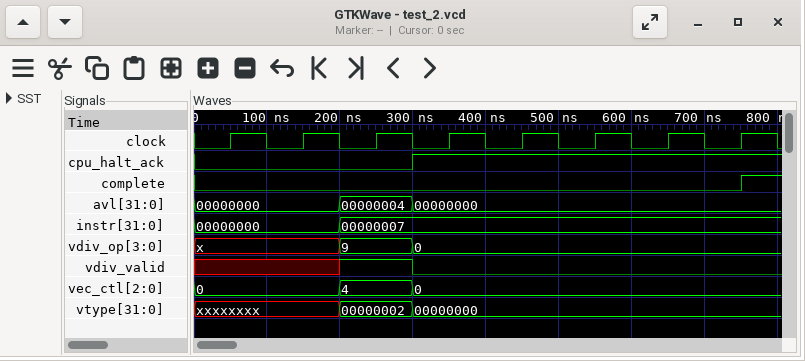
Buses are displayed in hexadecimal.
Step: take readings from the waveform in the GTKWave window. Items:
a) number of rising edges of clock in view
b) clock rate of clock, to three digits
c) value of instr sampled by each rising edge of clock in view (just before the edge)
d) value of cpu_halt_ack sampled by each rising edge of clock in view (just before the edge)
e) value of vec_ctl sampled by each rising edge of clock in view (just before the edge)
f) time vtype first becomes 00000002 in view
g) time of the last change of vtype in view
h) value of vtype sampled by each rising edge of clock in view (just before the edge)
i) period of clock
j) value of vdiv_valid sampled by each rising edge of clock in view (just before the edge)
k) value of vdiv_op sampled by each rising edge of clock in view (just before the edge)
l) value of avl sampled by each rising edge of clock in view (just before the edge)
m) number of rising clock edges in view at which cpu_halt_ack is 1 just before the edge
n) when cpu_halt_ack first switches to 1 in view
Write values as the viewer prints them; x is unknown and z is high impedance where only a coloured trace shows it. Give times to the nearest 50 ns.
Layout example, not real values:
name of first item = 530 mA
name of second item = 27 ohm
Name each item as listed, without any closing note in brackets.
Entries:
number of rising edges of clock in view = 8
clock rate of clock, to three digits = 10.0 MHz
value of instr sampled by each rising edge of clock in view = 00000000, 00000000, 00000007, 00000007, 00000007, 00000007, 00000007, 00000007
value of cpu_halt_ack sampled by each rising edge of clock in view = 0 0 0 1 1 1 1 1
value of vec_ctl sampled by each rising edge of clock in view = 0, 0, 4, 0, 0, 0, 0, 0
time vtype first becomes 00000002 in view = 200 ns
time of the last change of vtype in view = 300 ns
value of vtype sampled by each rising edge of clock in view = xxxxxxxx, xxxxxxxx, 00000002, 00000000, 00000000, 00000000, 00000000, 00000000
period of clock = 100 ns
value of vdiv_valid sampled by each rising edge of clock in view = x x 1 0 0 0 0 0
value of vdiv_op sampled by each rising edge of clock in view = x, x, 9, 0, 0, 0, 0, 0
value of avl sampled by each rising edge of clock in view = 00000000, 00000000, 00000004, 00000000, 00000000, 00000000, 00000000, 00000000
number of rising clock edges in view at which cpu_halt_ack is 1 just before the edge = 5
when cpu_halt_ack first switches to 1 in view = 300 ns
